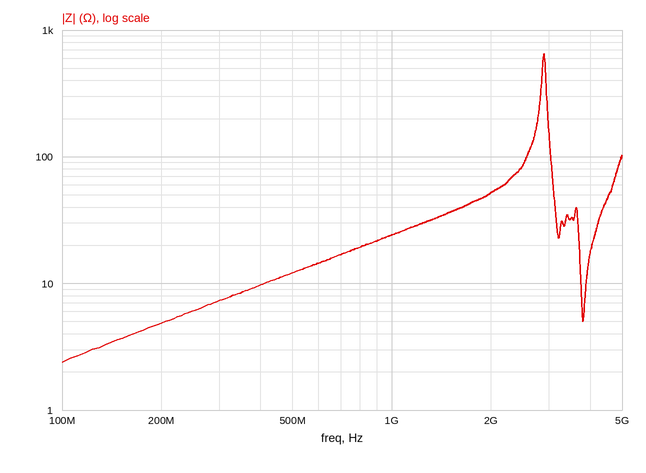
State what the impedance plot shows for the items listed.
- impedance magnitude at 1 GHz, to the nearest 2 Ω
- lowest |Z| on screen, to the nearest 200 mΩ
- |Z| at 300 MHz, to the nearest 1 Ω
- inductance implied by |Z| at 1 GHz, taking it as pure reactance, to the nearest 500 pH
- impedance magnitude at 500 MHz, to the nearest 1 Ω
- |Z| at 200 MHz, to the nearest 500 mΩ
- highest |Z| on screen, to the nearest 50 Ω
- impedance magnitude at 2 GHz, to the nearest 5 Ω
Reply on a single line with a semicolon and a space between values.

24 Ω; 2.4 Ω; 7 Ω; 4.0 nH; 12 Ω; 5.0 Ω; 650 Ω; 50 Ω
